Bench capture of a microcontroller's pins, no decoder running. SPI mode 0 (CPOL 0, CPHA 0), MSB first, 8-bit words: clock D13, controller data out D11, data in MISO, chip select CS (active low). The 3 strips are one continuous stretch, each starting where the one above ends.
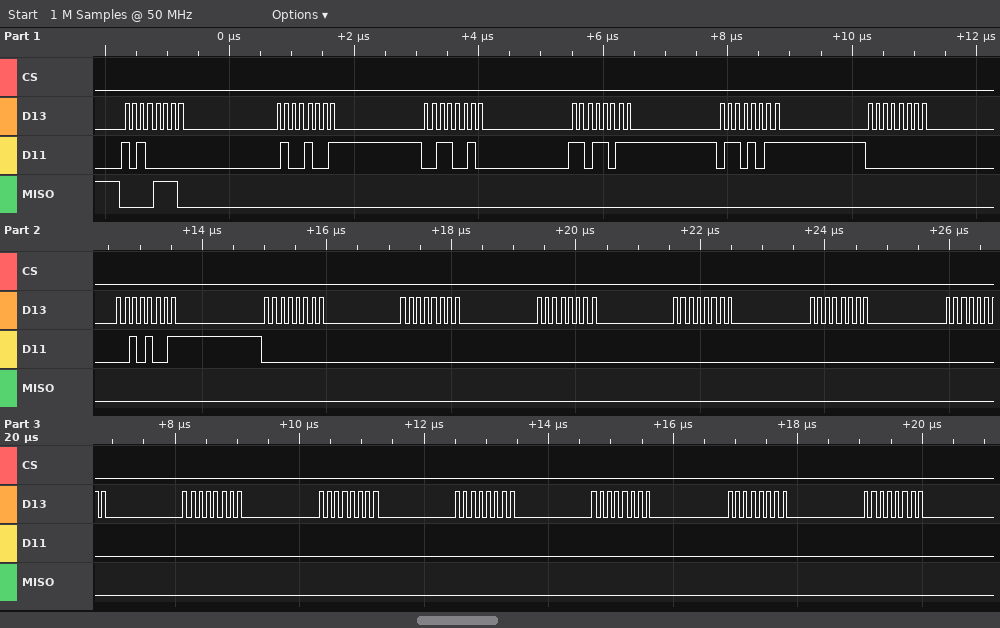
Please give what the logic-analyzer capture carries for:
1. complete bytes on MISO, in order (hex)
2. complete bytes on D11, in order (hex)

0E 00 00 00 00 00 00 00 00 00 00 00 00 00 00 00 00 00 00
A0 49 32 DB 6B 00 29 00 00 00 00 00 00 00 00 00 00 00 00
